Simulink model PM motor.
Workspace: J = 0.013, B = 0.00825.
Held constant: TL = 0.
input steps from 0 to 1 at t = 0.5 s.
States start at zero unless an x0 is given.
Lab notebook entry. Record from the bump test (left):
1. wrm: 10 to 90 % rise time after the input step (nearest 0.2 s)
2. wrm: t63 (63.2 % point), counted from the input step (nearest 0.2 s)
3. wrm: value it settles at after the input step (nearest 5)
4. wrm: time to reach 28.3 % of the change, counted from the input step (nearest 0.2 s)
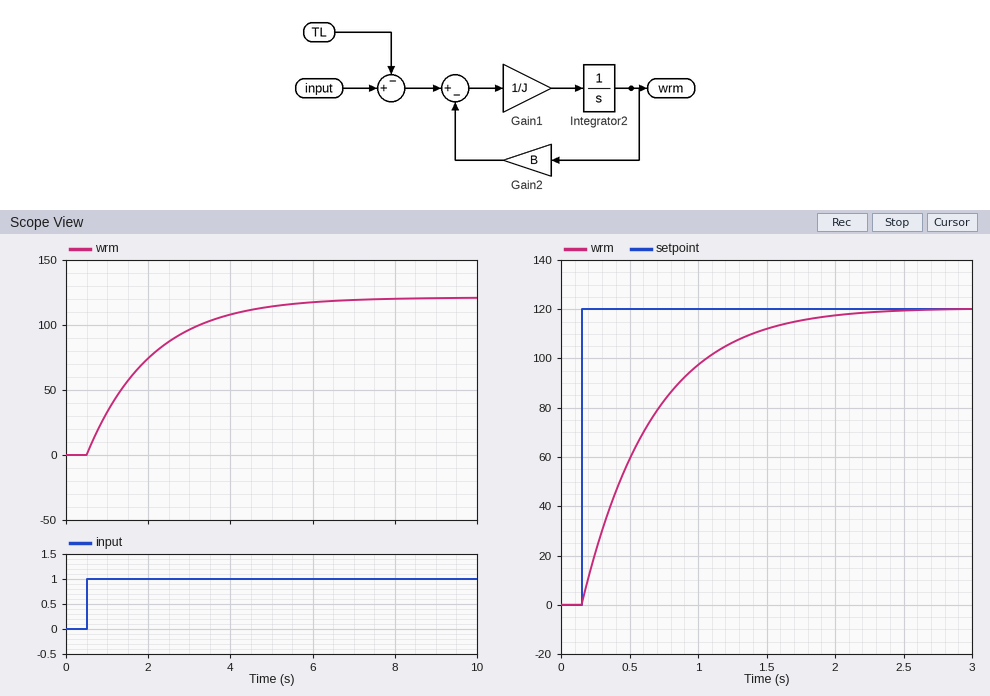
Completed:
3.4 s
1.6 s
120
0.6 s
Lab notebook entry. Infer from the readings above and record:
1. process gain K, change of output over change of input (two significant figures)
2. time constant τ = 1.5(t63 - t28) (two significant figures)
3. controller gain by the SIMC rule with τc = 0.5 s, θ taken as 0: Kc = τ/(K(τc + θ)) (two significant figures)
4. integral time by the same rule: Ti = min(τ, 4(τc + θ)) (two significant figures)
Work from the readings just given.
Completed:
120
1.5 s
0.025
1.5 s
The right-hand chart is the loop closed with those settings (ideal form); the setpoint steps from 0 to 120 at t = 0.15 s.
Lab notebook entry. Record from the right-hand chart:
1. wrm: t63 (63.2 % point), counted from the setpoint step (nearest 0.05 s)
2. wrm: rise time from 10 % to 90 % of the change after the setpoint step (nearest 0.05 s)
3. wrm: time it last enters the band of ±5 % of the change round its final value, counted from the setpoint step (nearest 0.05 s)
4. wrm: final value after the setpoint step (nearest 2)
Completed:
0.50 s
1.10 s
1.50 s
120
